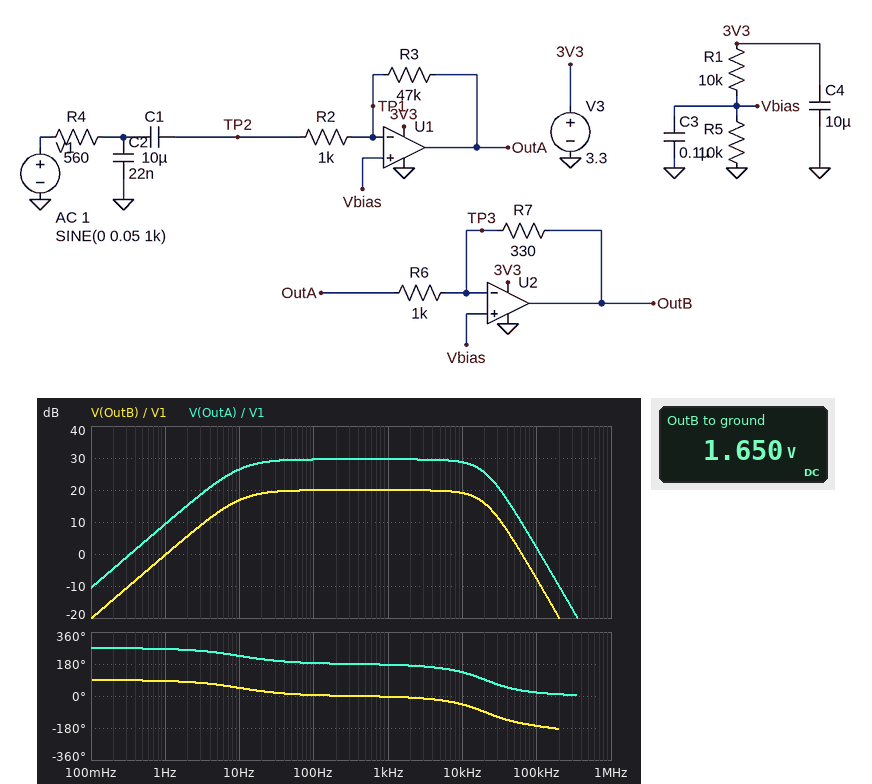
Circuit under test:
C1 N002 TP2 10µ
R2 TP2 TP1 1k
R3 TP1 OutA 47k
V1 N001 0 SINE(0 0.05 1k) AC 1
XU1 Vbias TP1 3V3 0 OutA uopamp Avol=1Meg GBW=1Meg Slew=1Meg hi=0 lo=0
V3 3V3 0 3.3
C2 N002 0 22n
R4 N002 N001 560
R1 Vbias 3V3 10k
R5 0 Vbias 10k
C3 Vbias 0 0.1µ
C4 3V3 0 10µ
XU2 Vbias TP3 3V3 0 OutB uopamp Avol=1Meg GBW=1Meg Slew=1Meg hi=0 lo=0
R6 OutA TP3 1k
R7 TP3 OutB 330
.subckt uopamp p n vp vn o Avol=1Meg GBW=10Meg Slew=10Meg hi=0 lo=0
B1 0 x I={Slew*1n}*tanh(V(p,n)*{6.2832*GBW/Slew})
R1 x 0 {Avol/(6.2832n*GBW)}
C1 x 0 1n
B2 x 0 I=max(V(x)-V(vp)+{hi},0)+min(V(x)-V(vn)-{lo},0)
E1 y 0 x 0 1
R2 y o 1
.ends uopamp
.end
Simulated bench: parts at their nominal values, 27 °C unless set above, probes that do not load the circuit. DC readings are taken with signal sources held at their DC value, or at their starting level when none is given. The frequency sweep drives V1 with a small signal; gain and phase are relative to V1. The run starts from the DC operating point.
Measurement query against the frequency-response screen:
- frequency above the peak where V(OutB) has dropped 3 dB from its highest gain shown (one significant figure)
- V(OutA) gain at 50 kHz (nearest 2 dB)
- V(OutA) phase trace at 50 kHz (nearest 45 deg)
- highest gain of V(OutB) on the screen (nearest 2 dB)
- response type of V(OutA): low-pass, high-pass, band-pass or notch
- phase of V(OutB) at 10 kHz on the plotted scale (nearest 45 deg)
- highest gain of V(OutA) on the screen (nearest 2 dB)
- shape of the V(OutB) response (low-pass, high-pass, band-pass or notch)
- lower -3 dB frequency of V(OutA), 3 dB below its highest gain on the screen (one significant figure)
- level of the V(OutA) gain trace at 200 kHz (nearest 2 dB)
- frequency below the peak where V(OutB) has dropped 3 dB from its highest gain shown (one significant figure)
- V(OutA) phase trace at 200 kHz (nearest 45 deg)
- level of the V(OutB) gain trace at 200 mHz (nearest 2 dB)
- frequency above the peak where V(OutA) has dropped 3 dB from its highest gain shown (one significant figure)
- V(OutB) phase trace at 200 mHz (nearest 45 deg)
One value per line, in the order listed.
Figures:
20 kHz
14 dB
45 deg
20 dB
band-pass
-45 deg
30 dB
band-pass
10 Hz
-10 dB
10 Hz
0 deg
-14 dB
20 kHz
90 deg
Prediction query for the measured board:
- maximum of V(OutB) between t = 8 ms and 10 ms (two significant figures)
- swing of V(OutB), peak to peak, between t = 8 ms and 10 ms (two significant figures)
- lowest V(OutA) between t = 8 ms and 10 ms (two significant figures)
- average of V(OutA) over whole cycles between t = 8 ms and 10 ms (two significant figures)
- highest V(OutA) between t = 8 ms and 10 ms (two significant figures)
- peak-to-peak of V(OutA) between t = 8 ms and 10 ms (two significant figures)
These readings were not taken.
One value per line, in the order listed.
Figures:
2.1 V
990 mV
150 mV
1.7 V
3.2 V
3.0 V
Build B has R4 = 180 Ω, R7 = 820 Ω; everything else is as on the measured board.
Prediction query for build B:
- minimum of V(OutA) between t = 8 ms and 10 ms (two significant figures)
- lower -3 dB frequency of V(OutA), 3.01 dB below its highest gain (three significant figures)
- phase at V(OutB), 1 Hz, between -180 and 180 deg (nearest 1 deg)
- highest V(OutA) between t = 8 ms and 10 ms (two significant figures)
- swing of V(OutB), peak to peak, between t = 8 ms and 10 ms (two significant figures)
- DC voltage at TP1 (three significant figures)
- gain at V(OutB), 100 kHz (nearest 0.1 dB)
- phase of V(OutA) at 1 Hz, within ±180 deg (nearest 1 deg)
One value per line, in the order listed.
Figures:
1.6 mV
13.5 Hz
86 deg
3.3 V
2.7 V
1.65 V
9.3 dB
-94 deg
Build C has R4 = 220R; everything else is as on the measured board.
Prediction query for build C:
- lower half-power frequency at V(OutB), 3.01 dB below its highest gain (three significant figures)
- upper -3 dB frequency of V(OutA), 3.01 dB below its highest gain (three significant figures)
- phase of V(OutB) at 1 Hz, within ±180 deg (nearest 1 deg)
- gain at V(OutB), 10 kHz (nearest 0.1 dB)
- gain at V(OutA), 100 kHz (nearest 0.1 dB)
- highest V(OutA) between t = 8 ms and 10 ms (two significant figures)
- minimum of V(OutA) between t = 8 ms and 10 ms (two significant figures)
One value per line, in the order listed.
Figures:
13.0 Hz
20.6 kHz
86 deg
21.3 dB
9.6 dB
3.3 V
1.6 mV
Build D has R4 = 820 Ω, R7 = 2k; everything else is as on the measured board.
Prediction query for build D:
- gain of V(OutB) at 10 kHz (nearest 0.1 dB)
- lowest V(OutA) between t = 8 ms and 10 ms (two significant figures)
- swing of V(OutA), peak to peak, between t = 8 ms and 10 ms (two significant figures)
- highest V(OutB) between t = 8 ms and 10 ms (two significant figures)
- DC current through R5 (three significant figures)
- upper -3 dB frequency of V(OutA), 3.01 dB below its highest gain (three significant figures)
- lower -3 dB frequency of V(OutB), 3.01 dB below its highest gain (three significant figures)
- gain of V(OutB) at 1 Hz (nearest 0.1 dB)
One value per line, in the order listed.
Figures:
33.2 dB
370 mV
2.6 V
3.3 V
165 µA
15.6 kHz
8.74 Hz
15.4 dB
